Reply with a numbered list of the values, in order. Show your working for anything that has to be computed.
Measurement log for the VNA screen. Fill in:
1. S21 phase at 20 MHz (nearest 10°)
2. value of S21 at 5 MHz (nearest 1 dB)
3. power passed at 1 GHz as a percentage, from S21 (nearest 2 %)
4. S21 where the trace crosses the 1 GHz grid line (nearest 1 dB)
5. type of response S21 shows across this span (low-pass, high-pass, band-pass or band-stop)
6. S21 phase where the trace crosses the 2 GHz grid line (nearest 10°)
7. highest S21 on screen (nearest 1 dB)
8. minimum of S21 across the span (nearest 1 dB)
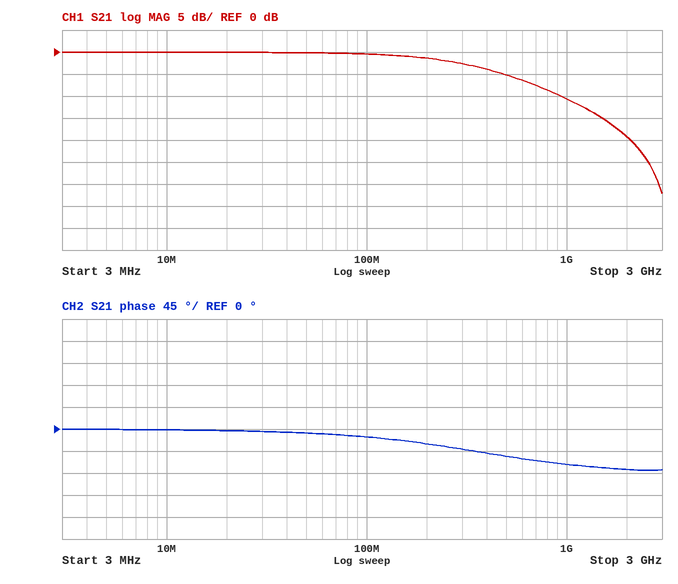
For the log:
1. 0°
2. 0 dB
3. 10^(-11/10) ≈ 8 %
4. -11 dB
5. low-pass
6. -80°
7. 0 dB
8. -32 dB
